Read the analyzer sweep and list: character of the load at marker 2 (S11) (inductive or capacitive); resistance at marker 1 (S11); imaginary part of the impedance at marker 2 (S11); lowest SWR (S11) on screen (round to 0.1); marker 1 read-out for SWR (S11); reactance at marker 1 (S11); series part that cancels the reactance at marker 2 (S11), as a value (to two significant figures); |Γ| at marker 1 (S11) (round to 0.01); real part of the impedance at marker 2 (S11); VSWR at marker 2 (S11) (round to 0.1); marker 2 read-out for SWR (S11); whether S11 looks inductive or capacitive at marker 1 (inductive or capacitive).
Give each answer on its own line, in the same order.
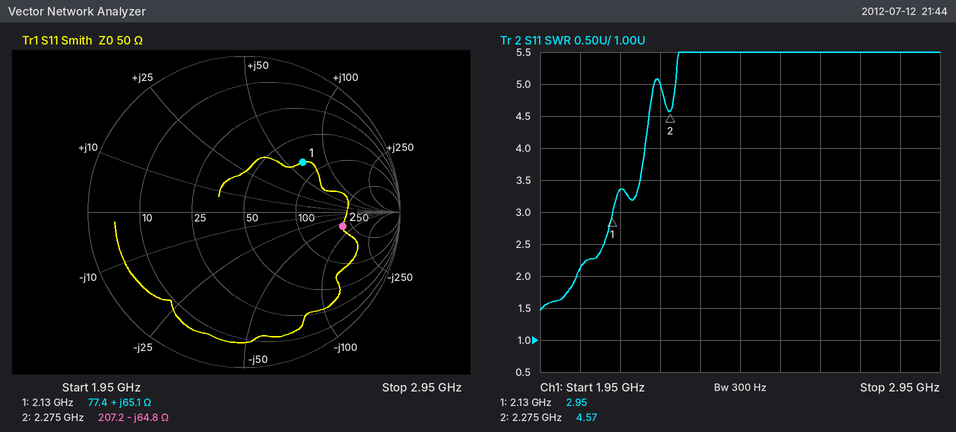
capacitive
77.4 Ω
-64.8 Ω
1.5
2.95
+65.1 Ω
4.5 nH
0.49
207.2 Ω
4.6
4.57
inductive
